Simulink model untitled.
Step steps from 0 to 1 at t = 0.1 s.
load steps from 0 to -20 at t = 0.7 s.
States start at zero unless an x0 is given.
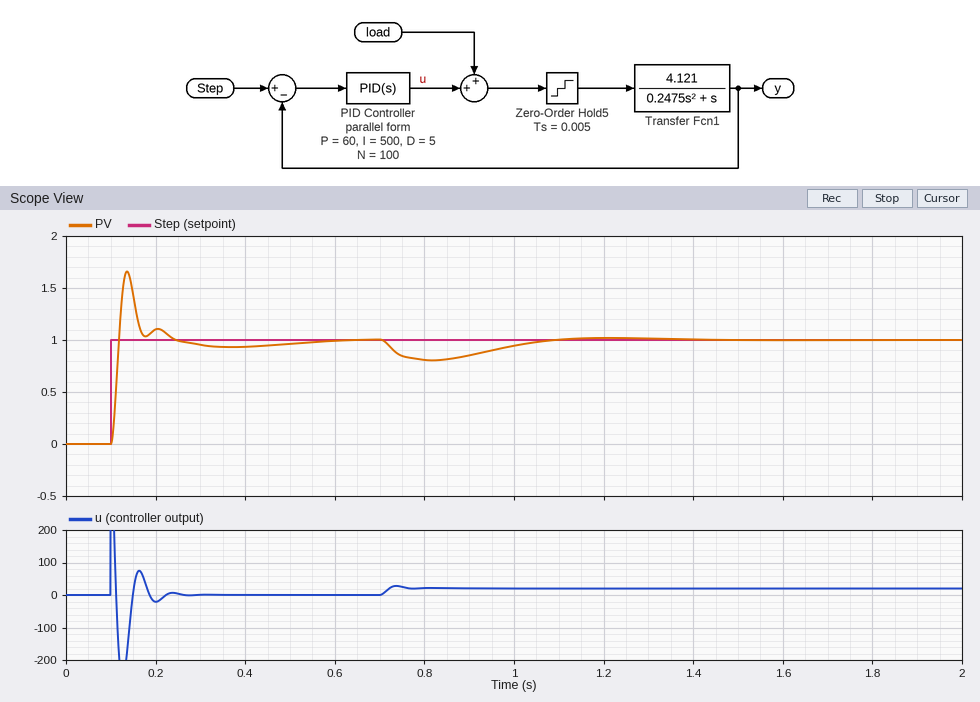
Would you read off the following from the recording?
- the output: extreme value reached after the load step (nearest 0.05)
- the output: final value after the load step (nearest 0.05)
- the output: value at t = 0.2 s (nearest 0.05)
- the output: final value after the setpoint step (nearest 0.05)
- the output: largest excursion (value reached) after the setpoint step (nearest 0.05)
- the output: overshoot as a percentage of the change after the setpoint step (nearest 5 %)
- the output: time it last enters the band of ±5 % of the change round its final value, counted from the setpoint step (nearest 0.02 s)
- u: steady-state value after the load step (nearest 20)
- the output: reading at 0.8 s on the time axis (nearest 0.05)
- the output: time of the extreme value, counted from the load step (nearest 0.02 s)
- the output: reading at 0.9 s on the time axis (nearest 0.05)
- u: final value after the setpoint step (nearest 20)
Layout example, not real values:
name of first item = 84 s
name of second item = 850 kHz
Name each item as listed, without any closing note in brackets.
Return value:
the output: extreme value reached after the load step = 0.80
the output: final value after the load step = 1.00
the output: value at t = 0.2 s = 1.10
the output: final value after the setpoint step = 1.00
the output: largest excursion (value reached) after the setpoint step = 1.65
the output: overshoot as a percentage of the change after the setpoint step = 65 %
the output: time it last enters the band of ±5 % of the change round its final value, counted from the setpoint step = 0.36 s
u: steady-state value after the load step = 20
the output: reading at 0.8 s on the time axis = 0.80
the output: time of the extreme value, counted from the load step = 0.12 s
the output: reading at 0.9 s on the time axis = 0.85
u: final value after the setpoint step = 0
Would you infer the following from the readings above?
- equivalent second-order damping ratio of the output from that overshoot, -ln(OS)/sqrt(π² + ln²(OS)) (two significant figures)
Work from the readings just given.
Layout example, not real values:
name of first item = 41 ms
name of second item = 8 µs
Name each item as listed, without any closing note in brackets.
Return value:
equivalent second-order damping ratio of the output from that overshoot, -ln(OS)/sqrt(π² + ln²(OS)) = 0.14
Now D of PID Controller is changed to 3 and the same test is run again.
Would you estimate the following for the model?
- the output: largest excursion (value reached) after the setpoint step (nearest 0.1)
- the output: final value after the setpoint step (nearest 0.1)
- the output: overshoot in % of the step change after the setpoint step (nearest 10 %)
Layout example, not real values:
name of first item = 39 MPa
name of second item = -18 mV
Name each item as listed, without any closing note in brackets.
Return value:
the output: largest excursion (value reached) after the setpoint step = 1.6
the output: final value after the setpoint step = 1.0
the output: overshoot in % of the step change after the setpoint step = 60 %
